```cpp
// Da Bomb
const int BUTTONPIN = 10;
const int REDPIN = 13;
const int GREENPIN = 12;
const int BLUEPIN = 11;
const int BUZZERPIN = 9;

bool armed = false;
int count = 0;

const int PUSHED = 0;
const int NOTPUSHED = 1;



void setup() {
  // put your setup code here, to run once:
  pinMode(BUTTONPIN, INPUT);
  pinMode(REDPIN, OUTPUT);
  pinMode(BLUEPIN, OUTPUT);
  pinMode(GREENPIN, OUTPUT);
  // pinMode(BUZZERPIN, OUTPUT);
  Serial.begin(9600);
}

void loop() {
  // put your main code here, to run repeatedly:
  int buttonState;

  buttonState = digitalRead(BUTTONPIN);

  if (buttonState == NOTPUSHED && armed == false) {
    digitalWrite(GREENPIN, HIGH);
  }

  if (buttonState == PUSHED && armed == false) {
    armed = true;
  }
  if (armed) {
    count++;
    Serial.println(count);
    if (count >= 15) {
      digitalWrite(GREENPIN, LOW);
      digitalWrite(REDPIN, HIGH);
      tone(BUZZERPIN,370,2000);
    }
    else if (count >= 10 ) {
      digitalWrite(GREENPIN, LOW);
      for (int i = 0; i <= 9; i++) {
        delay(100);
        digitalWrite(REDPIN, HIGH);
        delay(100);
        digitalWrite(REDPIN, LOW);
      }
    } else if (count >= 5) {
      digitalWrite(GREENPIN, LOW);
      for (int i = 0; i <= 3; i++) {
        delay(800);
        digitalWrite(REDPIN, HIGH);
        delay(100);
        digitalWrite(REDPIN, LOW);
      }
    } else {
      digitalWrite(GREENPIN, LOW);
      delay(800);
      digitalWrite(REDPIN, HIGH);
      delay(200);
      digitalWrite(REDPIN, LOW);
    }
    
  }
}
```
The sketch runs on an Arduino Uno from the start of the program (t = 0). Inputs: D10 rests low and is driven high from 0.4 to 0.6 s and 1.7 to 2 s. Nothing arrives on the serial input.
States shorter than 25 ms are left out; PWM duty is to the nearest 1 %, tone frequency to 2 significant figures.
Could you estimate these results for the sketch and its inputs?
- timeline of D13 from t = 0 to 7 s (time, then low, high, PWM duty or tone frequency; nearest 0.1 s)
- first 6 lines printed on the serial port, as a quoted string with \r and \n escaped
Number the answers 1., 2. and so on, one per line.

1. 0 s low; 0.8 s high; 1 s low; 1.8 s high; 2 s low; 2.8 s high; 3 s low; 3.8 s high; 4 s low; 4.8 s high; 4.9 s low; 5.7 s high; 5.8 s low; 6.6 s high; 6.7 s low
2. "1\r\n2\r\n3\r\n4\r\n5\r\n6\r\n"
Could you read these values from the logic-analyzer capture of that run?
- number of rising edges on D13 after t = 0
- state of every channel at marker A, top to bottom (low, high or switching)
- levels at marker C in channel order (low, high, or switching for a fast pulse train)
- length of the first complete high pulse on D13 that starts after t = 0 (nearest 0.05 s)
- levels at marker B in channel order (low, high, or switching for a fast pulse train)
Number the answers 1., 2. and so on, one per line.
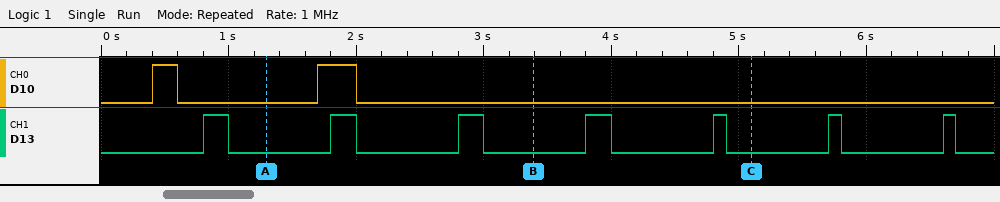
1. 7
2. D10 low, D13 low
3. D10 low, D13 low
4. 0.20 s
5. D10 low, D13 low
